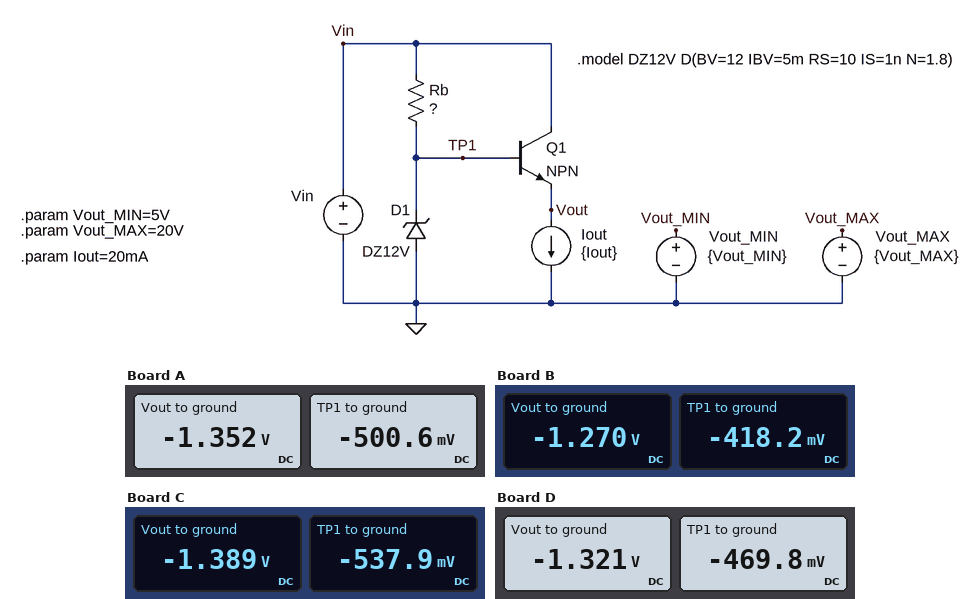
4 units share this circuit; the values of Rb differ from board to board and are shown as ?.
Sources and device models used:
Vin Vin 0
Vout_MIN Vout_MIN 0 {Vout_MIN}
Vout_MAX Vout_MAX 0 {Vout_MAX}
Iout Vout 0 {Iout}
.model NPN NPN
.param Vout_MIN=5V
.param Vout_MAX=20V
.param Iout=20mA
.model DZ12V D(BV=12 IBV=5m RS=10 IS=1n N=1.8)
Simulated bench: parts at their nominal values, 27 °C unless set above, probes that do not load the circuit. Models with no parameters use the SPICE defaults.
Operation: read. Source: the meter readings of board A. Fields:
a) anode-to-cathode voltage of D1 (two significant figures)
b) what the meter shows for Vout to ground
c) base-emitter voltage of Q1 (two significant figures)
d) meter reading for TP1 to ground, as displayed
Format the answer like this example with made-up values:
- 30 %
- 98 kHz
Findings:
- 500 mV
- -1.352 V
- 850 mV
- -500.6 mV
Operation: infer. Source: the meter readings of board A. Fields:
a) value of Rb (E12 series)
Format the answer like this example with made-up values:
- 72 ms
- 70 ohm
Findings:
- 3.3 kΩ
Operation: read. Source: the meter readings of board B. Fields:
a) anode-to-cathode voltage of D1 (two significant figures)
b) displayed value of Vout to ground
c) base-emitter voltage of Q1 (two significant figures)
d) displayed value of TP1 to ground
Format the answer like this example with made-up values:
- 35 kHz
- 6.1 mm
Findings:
- 420 mV
- -1.270 V
- 850 mV
- -418.2 mV
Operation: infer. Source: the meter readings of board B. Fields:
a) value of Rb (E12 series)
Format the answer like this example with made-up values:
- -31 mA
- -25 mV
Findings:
- 2.2 kΩ
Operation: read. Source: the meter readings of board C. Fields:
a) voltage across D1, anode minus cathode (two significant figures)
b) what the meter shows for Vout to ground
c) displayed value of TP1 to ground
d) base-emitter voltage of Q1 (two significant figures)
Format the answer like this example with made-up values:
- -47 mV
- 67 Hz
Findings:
- 540 mV
- -1.389 V
- -537.9 mV
- 850 mV
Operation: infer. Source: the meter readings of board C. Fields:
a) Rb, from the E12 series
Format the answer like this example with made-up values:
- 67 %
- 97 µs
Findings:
- 5.6 kΩ
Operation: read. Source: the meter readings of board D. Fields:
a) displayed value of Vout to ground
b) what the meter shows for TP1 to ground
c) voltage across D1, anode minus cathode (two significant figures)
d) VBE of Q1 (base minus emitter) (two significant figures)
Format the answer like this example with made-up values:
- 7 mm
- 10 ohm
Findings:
- -1.321 V
- -469.8 mV
- 470 mV
- 850 mV
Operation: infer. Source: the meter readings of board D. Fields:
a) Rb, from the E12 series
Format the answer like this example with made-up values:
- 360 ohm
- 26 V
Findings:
- 2.7 kΩ
